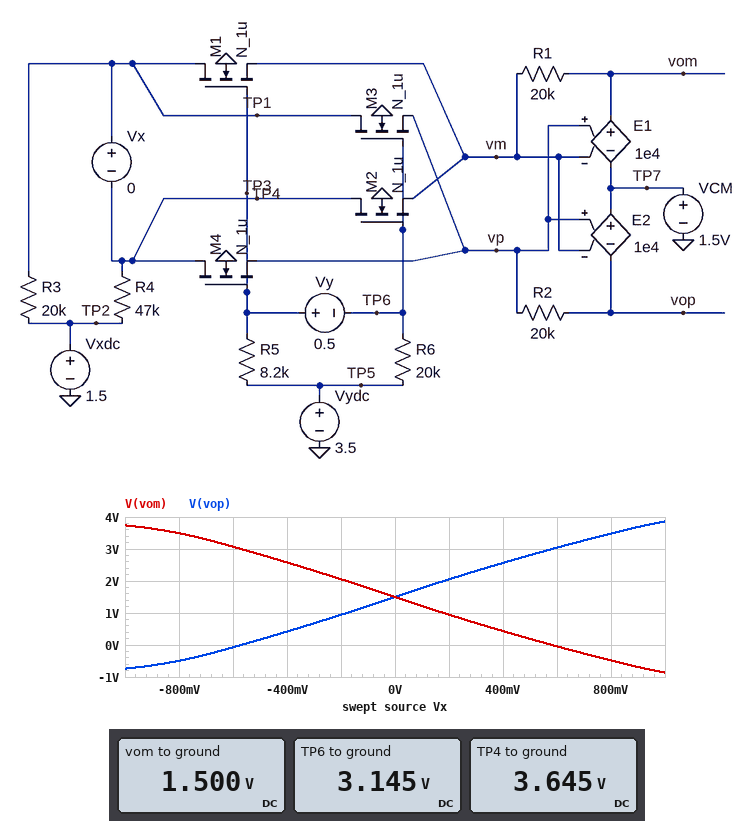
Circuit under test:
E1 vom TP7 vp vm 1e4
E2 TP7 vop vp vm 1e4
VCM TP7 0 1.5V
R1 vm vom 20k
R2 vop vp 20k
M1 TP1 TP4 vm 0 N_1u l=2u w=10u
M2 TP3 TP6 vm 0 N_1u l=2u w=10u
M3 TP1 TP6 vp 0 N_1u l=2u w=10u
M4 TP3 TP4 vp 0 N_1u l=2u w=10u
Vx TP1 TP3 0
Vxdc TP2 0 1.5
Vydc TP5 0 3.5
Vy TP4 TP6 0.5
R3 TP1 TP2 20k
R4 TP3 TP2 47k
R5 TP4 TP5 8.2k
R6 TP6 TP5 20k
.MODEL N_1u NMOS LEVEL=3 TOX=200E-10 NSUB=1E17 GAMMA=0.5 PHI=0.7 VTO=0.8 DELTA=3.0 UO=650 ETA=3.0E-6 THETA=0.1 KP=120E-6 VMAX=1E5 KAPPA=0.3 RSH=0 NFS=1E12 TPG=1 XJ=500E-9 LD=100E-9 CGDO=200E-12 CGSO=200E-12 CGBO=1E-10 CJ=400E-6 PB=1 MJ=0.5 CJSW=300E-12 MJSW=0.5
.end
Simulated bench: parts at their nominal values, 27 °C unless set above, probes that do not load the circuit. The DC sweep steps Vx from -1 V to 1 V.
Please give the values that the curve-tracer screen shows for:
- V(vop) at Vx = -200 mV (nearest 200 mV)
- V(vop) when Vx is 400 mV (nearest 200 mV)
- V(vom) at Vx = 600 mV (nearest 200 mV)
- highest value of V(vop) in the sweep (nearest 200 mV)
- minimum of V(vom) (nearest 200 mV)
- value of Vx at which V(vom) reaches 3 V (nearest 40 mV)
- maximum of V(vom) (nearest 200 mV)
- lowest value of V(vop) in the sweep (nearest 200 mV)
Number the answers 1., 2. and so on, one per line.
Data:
1. 1.0 V
2. 2.6 V
3. 0 V
4. 3.8 V
5. -800 mV
6. -560 mV
7. 3.8 V
8. -800 mV
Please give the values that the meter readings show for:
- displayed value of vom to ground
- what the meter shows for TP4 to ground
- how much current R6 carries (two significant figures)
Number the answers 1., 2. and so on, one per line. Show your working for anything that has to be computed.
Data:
1. 1.500 V
2. 3.645 V
3. (3.5 V - 3.145 V) / 20 kΩ = 18 µA
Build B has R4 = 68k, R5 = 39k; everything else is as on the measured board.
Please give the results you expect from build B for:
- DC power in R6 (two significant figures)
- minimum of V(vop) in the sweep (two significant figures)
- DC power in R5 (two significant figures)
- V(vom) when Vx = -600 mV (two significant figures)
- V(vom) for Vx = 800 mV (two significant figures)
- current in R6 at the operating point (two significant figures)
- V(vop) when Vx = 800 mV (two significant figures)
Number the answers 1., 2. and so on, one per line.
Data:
1. 1.4 µW
2. -850 mV
3. 2.8 µW
4. 3.0 V
5. -420 mV
6. 8.5 µA
7. 3.4 V
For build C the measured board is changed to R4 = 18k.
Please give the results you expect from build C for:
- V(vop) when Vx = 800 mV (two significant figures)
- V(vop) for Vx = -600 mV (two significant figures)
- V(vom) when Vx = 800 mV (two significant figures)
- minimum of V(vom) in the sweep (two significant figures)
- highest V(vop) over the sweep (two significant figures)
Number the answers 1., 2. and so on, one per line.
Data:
1. 3.5 V
2. -52 mV
3. -500 mV
4. -830 mV
5. 3.8 V
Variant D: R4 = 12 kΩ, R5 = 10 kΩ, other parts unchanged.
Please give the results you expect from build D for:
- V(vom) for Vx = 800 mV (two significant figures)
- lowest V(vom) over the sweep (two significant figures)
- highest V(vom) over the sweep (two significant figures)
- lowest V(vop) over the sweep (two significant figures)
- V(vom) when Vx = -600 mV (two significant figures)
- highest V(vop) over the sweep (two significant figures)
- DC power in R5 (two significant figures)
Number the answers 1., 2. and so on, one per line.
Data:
1. -500 mV
2. -810 mV
3. 3.9 V
4. -870 mV
5. 3.0 V
6. 3.8 V
7. 2.8 µW
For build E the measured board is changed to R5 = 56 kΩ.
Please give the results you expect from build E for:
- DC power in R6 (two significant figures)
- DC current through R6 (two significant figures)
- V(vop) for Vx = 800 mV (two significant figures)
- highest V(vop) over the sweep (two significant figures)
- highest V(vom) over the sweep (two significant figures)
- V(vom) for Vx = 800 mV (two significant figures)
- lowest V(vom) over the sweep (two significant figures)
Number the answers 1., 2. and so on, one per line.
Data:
1. 870 nW
2. 6.6 µA
3. 3.4 V
4. 3.8 V
5. 3.9 V
6. -420 mV
7. -820 mV
